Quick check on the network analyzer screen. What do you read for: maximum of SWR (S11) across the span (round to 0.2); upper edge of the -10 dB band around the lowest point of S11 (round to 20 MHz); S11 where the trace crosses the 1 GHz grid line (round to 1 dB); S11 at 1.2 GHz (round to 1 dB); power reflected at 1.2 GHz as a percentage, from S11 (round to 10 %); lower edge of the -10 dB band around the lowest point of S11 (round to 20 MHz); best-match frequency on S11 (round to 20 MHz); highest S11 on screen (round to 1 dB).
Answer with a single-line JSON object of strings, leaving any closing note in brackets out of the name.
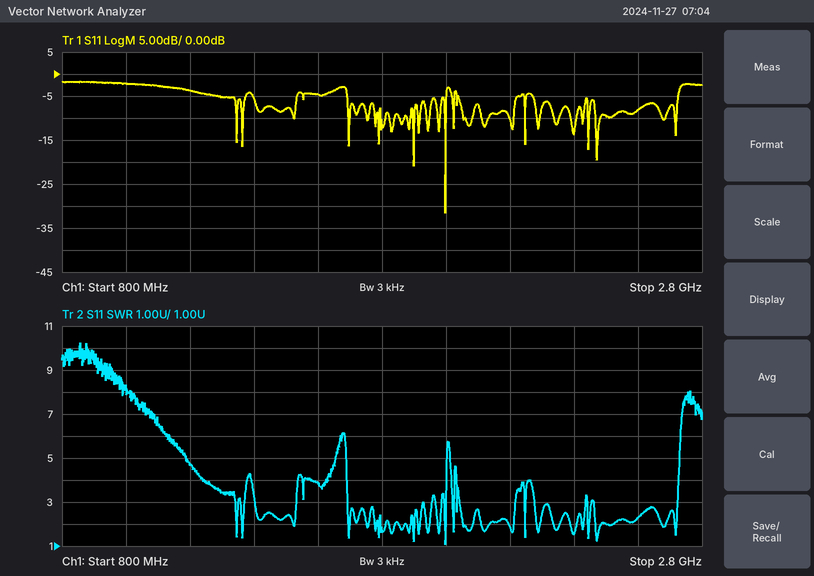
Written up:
{"maximum of SWR (S11) across the span": "10.2", "upper edge of the -10 dB band around the lowest point of S11": "2.00 GHz", "S11 where the trace crosses the 1 GHz grid line": "-2 dB", "S11 at 1.2 GHz": "-4 dB", "power reflected at 1.2 GHz as a percentage, from S11": "40 %", "lower edge of the -10 dB band around the lowest point of S11": "2.00 GHz", "best-match frequency on S11": "2.00 GHz", "highest S11 on screen": "-2 dB"}
